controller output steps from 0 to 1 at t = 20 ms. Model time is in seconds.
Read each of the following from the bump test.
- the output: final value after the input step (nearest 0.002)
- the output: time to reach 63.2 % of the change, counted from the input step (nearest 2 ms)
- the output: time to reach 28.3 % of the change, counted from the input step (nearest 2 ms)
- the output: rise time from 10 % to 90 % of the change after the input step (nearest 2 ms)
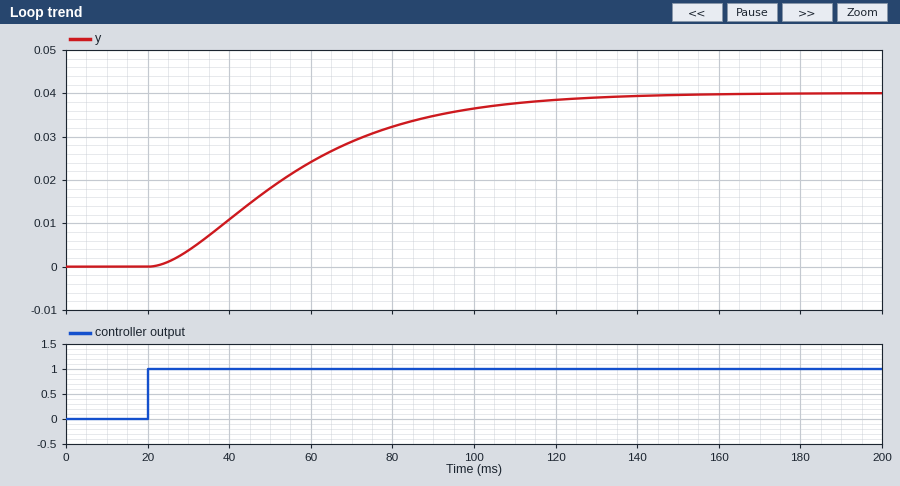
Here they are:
0.040
42 ms
20 ms
66 ms
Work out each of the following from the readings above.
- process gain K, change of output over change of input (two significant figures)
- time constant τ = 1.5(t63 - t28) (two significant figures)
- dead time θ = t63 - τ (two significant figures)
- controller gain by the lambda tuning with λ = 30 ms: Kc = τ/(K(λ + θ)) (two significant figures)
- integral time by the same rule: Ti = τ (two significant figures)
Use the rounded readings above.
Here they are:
0.040
33 ms
9.0 ms
21
33 ms
